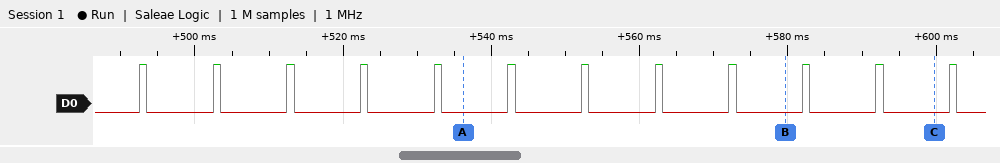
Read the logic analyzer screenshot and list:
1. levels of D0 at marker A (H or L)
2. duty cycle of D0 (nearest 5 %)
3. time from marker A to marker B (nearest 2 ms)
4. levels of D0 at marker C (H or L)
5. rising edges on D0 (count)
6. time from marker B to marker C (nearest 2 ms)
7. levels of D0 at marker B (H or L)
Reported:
D0=L
10 %
44 ms
D0=L
12
20 ms
D0=L
